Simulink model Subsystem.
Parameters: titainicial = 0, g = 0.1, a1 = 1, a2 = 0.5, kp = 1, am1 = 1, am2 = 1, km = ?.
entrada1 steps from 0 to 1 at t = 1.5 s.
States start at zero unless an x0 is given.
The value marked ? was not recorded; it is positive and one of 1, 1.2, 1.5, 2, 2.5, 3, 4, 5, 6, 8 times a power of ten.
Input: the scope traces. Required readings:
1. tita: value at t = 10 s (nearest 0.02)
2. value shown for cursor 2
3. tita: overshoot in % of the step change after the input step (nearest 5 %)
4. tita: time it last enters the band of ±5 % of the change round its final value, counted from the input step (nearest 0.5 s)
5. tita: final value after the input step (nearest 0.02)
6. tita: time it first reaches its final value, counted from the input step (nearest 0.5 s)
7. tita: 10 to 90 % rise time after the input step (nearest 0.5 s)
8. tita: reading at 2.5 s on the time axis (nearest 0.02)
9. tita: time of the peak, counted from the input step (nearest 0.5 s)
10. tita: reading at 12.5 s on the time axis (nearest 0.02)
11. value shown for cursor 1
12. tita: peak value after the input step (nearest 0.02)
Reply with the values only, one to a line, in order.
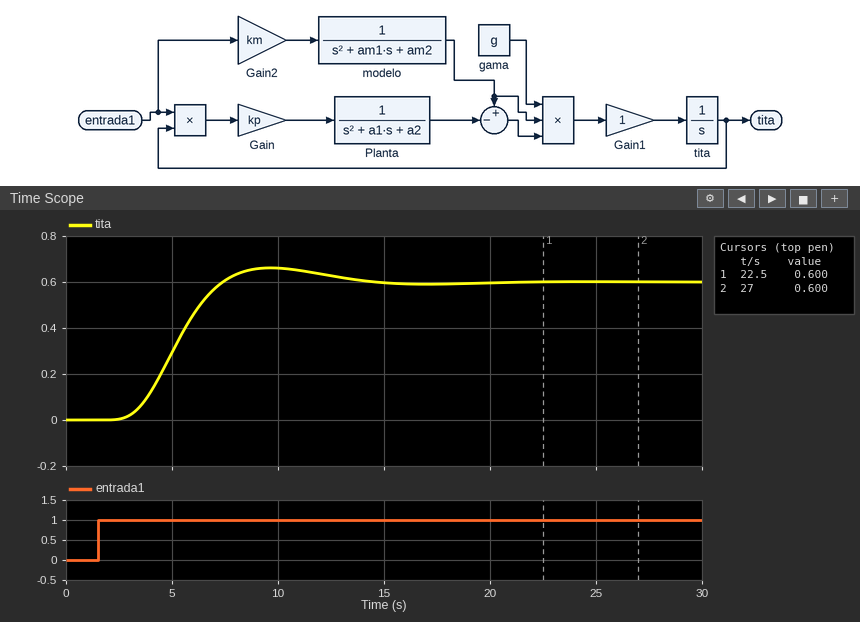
0.66
0.600
10 %
11.0 s
0.60
6.0 s
3.0 s
0.00
8.0 s
0.62
0.600
0.66
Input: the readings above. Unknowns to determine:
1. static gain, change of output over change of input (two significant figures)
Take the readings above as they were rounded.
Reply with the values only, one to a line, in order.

0.60
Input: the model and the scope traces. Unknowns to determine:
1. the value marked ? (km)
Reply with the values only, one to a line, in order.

1.2
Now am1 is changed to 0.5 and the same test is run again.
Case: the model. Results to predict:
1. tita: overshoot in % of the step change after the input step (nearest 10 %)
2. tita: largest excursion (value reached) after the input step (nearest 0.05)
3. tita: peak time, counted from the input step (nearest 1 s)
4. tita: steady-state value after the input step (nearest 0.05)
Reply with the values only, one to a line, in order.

30 %
0.75
6 s
0.60
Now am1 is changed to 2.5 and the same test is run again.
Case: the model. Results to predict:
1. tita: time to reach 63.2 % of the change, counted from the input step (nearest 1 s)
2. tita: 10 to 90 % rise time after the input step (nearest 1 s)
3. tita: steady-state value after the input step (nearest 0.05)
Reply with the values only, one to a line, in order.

6 s
6 s
0.60
